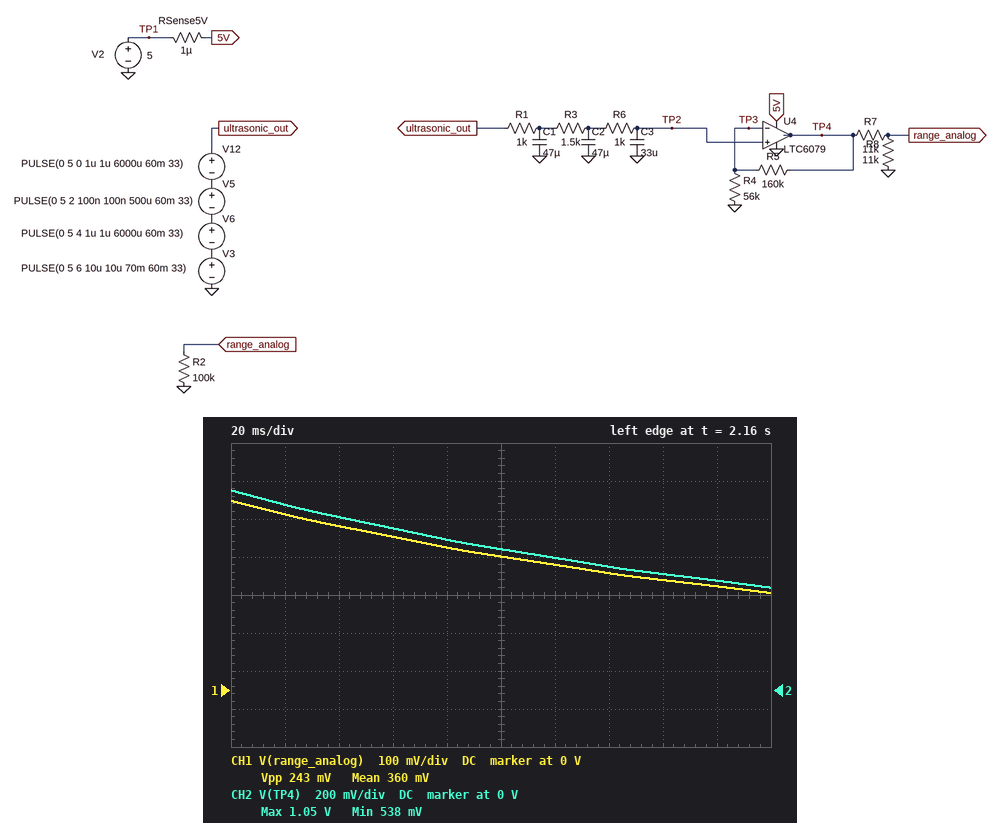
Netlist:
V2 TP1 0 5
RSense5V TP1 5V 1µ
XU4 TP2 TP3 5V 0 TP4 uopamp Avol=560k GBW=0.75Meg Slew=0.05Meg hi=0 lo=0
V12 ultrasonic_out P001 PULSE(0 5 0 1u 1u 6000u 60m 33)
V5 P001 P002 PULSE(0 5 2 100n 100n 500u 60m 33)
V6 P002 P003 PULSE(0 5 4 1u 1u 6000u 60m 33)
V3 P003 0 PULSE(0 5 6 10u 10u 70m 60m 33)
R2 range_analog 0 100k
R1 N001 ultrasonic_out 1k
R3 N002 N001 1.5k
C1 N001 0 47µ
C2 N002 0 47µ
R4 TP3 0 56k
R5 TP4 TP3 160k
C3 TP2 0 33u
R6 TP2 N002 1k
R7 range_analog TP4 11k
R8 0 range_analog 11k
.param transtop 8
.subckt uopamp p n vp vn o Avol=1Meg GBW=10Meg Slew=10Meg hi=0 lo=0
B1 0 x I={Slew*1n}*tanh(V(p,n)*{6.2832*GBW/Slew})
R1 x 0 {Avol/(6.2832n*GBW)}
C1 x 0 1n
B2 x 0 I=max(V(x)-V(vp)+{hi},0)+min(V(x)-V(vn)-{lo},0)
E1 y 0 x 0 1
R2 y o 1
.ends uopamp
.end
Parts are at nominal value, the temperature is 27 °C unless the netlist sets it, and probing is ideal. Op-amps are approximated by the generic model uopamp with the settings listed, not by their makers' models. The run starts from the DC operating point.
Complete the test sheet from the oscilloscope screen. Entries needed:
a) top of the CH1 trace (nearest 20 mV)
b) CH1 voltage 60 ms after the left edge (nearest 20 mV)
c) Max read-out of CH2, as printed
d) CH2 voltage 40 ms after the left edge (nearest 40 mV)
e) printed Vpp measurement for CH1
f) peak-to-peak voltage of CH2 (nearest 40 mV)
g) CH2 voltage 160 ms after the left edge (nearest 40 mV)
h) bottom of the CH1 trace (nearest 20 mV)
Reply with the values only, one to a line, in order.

500 mV
400 mV
1.05 V
920 mV
243 mV
520 mV
600 mV
260 mV
